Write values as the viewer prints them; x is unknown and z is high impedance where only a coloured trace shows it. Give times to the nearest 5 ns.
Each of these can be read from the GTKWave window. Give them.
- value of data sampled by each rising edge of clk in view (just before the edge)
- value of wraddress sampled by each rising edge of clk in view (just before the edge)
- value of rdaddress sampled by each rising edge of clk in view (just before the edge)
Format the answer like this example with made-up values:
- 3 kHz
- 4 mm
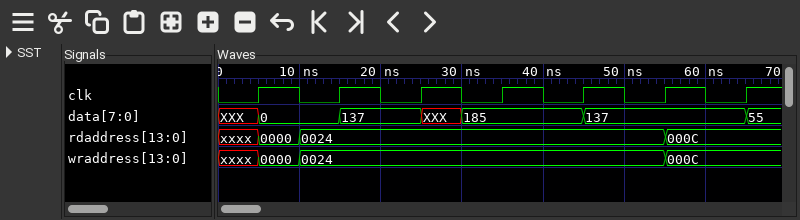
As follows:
- XXX, 0, 137, 185, 185, 137, 137
- xxxx, 0024, 0024, 0024, 0024, 0024, 000C
- xxxx, 0024, 0024, 0024, 0024, 0024, 000C
